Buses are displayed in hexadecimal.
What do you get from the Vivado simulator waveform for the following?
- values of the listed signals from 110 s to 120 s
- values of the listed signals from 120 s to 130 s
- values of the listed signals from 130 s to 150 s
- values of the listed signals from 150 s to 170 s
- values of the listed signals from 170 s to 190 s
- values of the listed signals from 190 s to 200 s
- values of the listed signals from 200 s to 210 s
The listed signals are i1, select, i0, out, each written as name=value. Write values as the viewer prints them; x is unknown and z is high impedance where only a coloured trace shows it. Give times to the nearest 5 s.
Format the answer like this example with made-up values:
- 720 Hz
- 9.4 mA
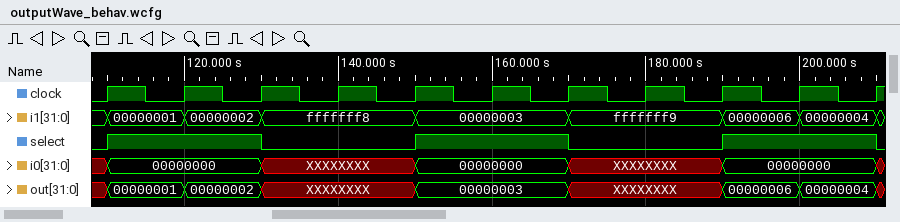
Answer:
- i1=00000001, select=1, i0=00000000, out=00000001
- i1=00000002, select=1, i0=00000000, out=00000002
- i1=fffffff8, select=0, i0=XXXXXXXX, out=XXXXXXXX
- i1=00000003, select=1, i0=00000000, out=00000003
- i1=fffffff9, select=0, i0=XXXXXXXX, out=XXXXXXXX
- i1=00000006, select=1, i0=00000000, out=00000006
- i1=00000004, select=1, i0=00000000, out=00000004
